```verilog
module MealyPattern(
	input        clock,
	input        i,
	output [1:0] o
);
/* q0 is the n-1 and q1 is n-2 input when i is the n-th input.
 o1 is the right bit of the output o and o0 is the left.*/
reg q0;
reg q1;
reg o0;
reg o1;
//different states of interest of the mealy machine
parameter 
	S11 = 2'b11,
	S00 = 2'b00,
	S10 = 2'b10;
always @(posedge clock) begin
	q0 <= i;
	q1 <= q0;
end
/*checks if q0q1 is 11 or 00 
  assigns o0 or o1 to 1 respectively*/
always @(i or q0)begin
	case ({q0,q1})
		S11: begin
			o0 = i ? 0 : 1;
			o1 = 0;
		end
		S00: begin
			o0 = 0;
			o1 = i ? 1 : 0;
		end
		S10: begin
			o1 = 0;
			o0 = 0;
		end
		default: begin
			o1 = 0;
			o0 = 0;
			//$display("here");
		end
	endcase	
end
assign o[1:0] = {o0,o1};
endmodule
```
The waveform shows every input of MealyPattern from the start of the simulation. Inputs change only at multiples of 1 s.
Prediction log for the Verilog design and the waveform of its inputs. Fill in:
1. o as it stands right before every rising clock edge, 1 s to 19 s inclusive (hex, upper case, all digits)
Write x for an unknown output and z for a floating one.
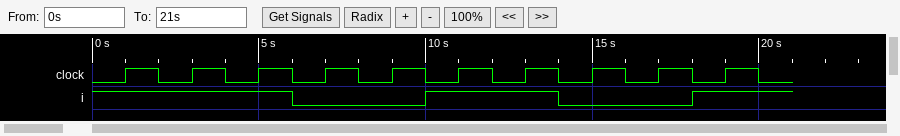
0, 0, 0, 2, 0, 1, 0, 2, 0, 1
